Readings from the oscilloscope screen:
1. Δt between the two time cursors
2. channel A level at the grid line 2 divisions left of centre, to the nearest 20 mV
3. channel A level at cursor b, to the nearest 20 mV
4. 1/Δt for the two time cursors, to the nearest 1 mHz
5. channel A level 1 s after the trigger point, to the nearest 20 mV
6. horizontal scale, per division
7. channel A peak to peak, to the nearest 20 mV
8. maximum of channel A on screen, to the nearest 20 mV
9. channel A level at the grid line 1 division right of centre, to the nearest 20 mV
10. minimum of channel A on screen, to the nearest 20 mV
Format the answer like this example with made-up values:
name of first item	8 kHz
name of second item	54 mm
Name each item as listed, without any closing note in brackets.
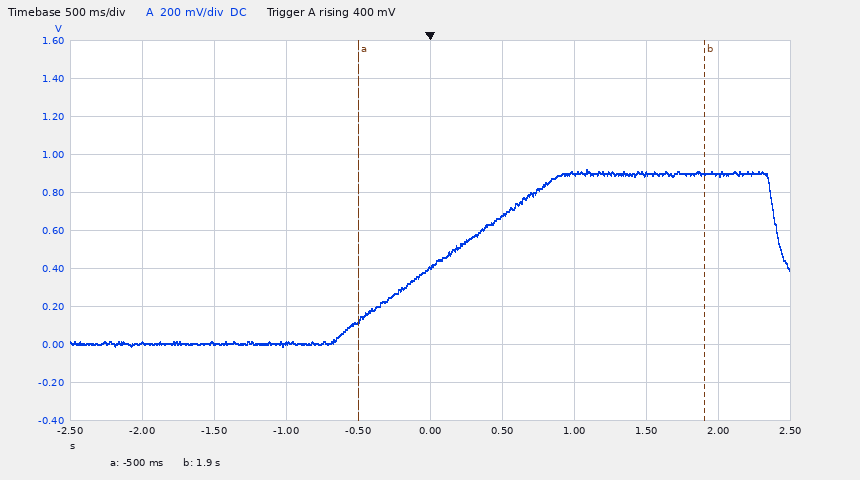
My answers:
Δt between the two time cursors	2.40 s
channel A level at the grid line 2 divisions left of centre, to the nearest 20 mV	0 mV
channel A level at cursor b, to the nearest 20 mV	900 mV
1/Δt for the two time cursors, to the nearest 1 mHz	417 mHz
channel A level 1 s after the trigger point, to the nearest 20 mV	900 mV
horizontal scale, per division	500 ms
channel A peak to peak, to the nearest 20 mV	940 mV
maximum of channel A on screen, to the nearest 20 mV	920 mV
channel A level at the grid line 1 division right of centre, to the nearest 20 mV	680 mV
minimum of channel A on screen, to the nearest 20 mV	-20 mV
